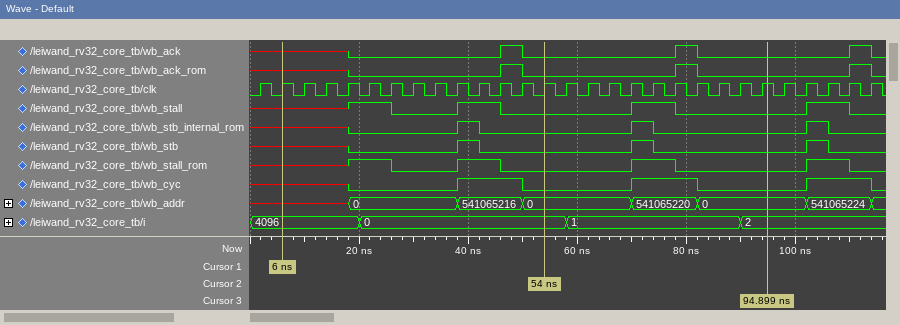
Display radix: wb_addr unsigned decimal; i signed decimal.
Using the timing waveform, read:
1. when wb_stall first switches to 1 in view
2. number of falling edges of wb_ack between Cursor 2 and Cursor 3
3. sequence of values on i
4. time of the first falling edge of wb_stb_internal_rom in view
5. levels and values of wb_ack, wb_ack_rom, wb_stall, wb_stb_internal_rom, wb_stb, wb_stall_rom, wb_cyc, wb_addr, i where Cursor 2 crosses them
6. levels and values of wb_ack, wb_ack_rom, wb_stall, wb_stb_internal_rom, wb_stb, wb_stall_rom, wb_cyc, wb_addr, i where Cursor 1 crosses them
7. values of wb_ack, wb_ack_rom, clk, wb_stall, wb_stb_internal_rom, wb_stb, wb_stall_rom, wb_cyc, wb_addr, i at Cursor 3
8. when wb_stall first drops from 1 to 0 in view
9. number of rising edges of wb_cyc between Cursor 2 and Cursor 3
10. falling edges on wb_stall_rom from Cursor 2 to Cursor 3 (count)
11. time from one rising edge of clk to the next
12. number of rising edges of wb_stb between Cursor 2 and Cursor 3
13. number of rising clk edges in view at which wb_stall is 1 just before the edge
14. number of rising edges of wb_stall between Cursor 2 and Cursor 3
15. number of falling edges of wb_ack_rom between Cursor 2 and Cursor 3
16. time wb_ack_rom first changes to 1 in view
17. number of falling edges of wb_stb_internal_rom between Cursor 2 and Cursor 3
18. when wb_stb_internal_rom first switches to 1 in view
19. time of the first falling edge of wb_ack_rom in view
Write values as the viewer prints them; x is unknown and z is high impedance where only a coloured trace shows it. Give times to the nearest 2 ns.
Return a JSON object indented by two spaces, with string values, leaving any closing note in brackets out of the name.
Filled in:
{
  "when wb_stall first switches to 1 in view": "18 ns",
  "number of falling edges of wb_ack between Cursor 2 and Cursor 3": "1",
  "sequence of values on i": "4096, 0, 1, 2",
  "time of the first falling edge of wb_stb_internal_rom in view": "42 ns",
  "levels and values of wb_ack, wb_ack_rom, wb_stall, wb_stb_internal_rom, wb_stb, wb_stall_rom, wb_cyc, wb_addr, i where Cursor 2 crosses them": "wb_ack=0, wb_ack_rom=0, wb_stall=0, wb_stb_internal_rom=0, wb_stb=0, wb_stall_rom=0, wb_cyc=0, wb_addr=0, i=0",
  "levels and values of wb_ack, wb_ack_rom, wb_stall, wb_stb_internal_rom, wb_stb, wb_stall_rom, wb_cyc, wb_addr, i where Cursor 1 crosses them": "wb_ack=x, wb_ack_rom=x, wb_stall=x, wb_stb_internal_rom=x, wb_stb=x, wb_stall_rom=x, wb_cyc=x, wb_addr=x, i=4096",
  "values of wb_ack, wb_ack_rom, clk, wb_stall, wb_stb_internal_rom, wb_stb, wb_stall_rom, wb_cyc, wb_addr, i at Cursor 3": "wb_ack=0, wb_ack_rom=0, clk=1, wb_stall=0, wb_stb_internal_rom=0, wb_stb=0, wb_stall_rom=0, wb_cyc=0, wb_addr=0, i=2",
  "when wb_stall first drops from 1 to 0 in view": "26 ns",
  "number of rising edges of wb_cyc between Cursor 2 and Cursor 3": "1",
  "falling edges on wb_stall_rom from Cursor 2 to Cursor 3": "1",
  "time from one rising edge of clk to the next": "4 ns",
  "number of rising edges of wb_stb between Cursor 2 and Cursor 3": "1",
  "number of rising clk edges in view at which wb_stall is 1 just before the edge": "8",
  "number of rising edges of wb_stall between Cursor 2 and Cursor 3": "1",
  "number of falling edges of wb_ack_rom between Cursor 2 and Cursor 3": "1",
  "time wb_ack_rom first changes to 1 in view": "46 ns",
  "number of falling edges of wb_stb_internal_rom between Cursor 2 and Cursor 3": "1",
  "when wb_stb_internal_rom first switches to 1 in view": "38 ns",
  "time of the first falling edge of wb_ack_rom in view": "50 ns"
}
